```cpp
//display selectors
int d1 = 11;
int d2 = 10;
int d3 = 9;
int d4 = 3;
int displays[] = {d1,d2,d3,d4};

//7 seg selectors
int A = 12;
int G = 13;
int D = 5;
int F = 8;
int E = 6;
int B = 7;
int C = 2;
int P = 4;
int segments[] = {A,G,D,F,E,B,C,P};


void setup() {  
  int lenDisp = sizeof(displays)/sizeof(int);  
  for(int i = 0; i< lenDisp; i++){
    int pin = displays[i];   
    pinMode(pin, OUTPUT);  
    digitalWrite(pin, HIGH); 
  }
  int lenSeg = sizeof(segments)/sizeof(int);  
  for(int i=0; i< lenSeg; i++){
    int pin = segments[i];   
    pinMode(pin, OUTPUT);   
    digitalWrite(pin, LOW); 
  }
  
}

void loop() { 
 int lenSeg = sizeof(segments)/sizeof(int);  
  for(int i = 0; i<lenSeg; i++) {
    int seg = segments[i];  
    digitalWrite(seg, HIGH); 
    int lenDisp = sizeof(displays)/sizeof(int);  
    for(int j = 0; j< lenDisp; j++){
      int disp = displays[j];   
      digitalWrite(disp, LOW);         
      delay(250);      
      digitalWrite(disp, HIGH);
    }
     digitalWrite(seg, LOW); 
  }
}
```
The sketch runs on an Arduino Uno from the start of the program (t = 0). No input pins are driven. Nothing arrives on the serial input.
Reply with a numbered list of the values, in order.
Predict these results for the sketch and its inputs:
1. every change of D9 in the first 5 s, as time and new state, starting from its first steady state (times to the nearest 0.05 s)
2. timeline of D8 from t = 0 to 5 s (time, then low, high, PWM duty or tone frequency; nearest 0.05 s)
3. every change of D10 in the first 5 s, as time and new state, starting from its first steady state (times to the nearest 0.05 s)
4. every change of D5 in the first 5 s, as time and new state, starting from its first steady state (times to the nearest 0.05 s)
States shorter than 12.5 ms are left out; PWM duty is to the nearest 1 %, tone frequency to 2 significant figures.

1. 0 s high; 0.5 s low; 0.75 s high; 1.5 s low; 1.75 s high; 2.5 s low; 2.75 s high; 3.5 s low; 3.75 s high; 4.5 s low; 4.75 s high
2. 0 s low; 3 s high; 4 s low
3. 0 s high; 0.25 s low; 0.5 s high; 1.25 s low; 1.5 s high; 2.25 s low; 2.5 s high; 3.25 s low; 3.5 s high; 4.25 s low; 4.5 s high
4. 0 s low; 2 s high; 3 s low
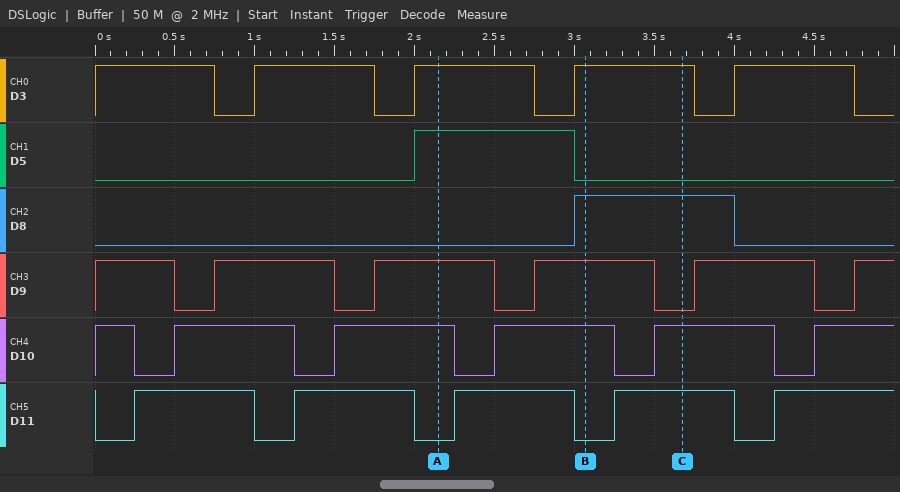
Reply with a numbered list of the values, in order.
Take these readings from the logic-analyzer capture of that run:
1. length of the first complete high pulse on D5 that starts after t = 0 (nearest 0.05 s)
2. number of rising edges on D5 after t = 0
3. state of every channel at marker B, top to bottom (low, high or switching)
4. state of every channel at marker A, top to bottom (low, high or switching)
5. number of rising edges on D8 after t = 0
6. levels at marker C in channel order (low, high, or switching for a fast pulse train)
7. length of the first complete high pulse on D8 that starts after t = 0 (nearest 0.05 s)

1. 1.00 s
2. 1
3. D3 high, D5 low, D8 high, D9 high, D10 high, D11 low
4. D3 high, D5 high, D8 low, D9 high, D10 high, D11 low
5. 1
6. D3 high, D5 low, D8 high, D9 low, D10 high, D11 high
7. 1.00 s
